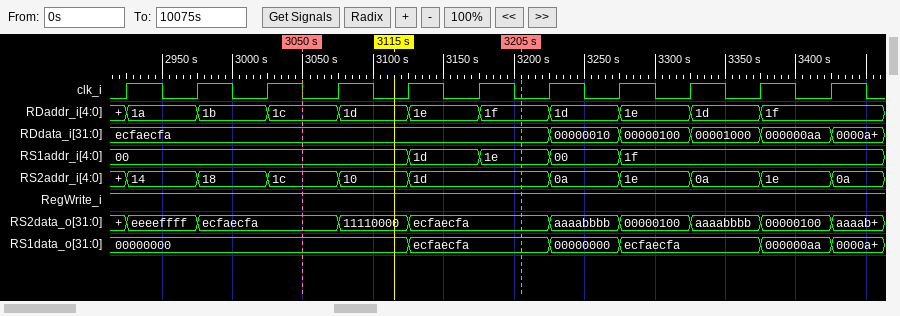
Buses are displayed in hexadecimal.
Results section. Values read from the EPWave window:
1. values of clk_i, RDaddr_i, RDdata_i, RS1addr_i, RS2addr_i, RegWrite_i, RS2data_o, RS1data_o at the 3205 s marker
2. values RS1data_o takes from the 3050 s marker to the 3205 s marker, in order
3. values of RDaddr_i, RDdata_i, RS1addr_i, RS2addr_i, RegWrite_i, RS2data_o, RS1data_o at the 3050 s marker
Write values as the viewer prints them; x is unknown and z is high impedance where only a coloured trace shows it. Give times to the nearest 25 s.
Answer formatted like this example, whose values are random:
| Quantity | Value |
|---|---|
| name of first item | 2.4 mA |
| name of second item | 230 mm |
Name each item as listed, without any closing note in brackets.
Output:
| Quantity | Value |
|---|---|
| values of clk_i, RDaddr_i, RDdata_i, RS1addr_i, RS2addr_i, RegWrite_i, RS2data_o, RS1data_o at the 3205 s marker | clk_i=0, RDaddr_i=1f, RDdata_i=ecfaecfa, RS1addr_i=1e, RS2addr_i=1d, RegWrite_i=1, RS2data_o=ecfaecfa, RS1data_o=ecfaecfa |
| values RS1data_o takes from the 3050 s marker to the 3205 s marker, in order | 00000000, ecfaecfa |
| values of RDaddr_i, RDdata_i, RS1addr_i, RS2addr_i, RegWrite_i, RS2data_o, RS1data_o at the 3050 s marker | RDaddr_i=1c, RDdata_i=ecfaecfa, RS1addr_i=00, RS2addr_i=1c, RegWrite_i=1, RS2data_o=ecfaecfa, RS1data_o=00000000 |
